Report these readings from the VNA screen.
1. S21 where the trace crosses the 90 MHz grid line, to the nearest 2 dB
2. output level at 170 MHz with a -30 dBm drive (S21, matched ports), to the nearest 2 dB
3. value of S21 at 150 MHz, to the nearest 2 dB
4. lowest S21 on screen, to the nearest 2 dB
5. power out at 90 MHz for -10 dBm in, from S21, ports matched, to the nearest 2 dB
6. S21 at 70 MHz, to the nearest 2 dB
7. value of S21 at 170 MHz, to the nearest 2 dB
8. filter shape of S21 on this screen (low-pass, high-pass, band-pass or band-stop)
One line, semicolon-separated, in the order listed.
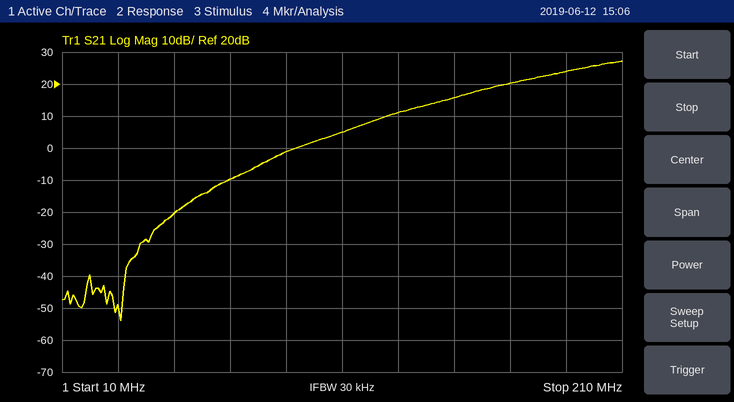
-2 dB; -10 dBm; 16 dB; -54 dB; -12 dBm; -10 dB; 20 dB; high-pass
